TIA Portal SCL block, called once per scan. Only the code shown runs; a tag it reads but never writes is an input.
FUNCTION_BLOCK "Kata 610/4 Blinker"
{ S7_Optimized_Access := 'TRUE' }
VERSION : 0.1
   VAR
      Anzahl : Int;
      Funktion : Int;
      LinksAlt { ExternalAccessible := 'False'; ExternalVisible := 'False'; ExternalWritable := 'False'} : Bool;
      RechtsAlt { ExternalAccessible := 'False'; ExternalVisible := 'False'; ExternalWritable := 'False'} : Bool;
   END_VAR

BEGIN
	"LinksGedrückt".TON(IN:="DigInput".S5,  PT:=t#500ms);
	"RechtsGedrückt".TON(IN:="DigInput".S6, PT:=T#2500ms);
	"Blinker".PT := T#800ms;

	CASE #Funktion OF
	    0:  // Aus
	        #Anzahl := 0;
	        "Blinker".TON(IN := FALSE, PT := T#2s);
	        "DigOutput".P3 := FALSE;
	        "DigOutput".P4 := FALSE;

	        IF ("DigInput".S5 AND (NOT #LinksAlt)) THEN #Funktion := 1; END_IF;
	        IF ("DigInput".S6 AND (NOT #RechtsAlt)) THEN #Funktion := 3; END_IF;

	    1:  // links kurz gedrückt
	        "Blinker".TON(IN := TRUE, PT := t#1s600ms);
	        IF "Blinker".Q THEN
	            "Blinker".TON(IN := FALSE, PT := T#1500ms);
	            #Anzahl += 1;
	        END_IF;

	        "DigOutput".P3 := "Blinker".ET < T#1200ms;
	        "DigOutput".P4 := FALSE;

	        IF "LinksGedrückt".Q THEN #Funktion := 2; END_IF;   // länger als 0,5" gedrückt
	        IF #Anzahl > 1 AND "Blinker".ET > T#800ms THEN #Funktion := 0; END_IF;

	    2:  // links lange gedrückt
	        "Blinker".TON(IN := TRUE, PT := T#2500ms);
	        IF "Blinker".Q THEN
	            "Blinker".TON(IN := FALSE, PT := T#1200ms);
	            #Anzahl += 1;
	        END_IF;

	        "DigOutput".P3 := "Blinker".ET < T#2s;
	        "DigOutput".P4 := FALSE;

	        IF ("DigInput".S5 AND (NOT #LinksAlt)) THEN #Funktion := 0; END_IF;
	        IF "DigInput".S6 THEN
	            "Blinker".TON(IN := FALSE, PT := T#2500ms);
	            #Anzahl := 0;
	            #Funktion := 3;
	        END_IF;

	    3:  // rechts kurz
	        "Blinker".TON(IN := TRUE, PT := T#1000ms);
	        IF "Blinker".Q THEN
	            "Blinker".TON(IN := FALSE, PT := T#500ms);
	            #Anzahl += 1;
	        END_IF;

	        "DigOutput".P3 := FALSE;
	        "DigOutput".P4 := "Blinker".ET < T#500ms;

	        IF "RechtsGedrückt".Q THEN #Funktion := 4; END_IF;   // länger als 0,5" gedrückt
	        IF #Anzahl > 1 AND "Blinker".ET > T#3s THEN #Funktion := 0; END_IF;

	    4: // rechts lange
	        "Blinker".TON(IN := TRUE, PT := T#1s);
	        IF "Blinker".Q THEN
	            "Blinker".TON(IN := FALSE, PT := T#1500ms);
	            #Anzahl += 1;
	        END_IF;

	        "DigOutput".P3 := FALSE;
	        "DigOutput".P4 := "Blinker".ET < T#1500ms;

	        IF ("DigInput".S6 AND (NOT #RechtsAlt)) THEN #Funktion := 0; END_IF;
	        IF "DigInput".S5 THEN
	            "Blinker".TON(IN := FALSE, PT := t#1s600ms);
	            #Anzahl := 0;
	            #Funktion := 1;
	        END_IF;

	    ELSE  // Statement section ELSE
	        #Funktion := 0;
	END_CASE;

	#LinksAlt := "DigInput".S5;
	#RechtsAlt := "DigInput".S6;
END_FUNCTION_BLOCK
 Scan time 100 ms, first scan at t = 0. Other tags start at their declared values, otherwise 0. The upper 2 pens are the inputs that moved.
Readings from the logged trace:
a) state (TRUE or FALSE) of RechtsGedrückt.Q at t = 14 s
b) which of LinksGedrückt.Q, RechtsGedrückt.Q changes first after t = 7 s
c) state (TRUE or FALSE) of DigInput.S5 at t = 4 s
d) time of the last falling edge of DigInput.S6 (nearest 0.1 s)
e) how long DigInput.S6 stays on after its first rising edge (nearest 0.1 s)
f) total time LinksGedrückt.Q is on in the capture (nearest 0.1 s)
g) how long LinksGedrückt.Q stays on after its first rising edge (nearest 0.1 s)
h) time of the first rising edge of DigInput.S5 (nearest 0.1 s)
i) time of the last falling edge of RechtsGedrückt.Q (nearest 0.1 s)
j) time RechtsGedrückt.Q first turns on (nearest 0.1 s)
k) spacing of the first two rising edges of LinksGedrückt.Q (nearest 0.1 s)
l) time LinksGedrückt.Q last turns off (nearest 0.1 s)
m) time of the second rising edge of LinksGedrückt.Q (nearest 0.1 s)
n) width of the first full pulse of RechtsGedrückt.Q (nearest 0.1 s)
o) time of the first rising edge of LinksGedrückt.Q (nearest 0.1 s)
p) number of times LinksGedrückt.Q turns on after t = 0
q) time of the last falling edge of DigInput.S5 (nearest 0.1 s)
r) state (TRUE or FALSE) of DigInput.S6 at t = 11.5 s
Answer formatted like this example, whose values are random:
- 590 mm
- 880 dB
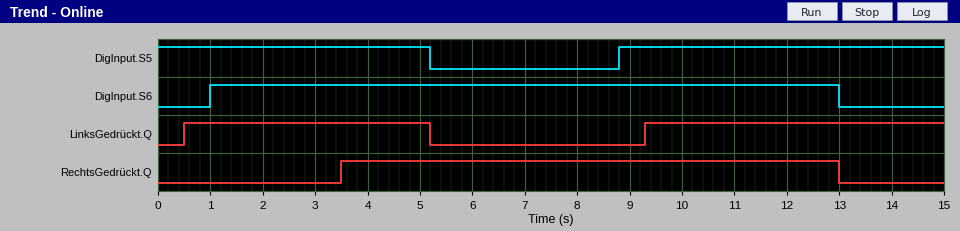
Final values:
- FALSE
- LinksGedrückt.Q
- TRUE
- 13.0 s
- 12.0 s
- 10.4 s
- 4.7 s
- 8.8 s
- 13.0 s
- 3.5 s
- 8.8 s
- 5.2 s
- 9.3 s
- 9.5 s
- 0.5 s
- 2
- 5.2 s
- TRUE
